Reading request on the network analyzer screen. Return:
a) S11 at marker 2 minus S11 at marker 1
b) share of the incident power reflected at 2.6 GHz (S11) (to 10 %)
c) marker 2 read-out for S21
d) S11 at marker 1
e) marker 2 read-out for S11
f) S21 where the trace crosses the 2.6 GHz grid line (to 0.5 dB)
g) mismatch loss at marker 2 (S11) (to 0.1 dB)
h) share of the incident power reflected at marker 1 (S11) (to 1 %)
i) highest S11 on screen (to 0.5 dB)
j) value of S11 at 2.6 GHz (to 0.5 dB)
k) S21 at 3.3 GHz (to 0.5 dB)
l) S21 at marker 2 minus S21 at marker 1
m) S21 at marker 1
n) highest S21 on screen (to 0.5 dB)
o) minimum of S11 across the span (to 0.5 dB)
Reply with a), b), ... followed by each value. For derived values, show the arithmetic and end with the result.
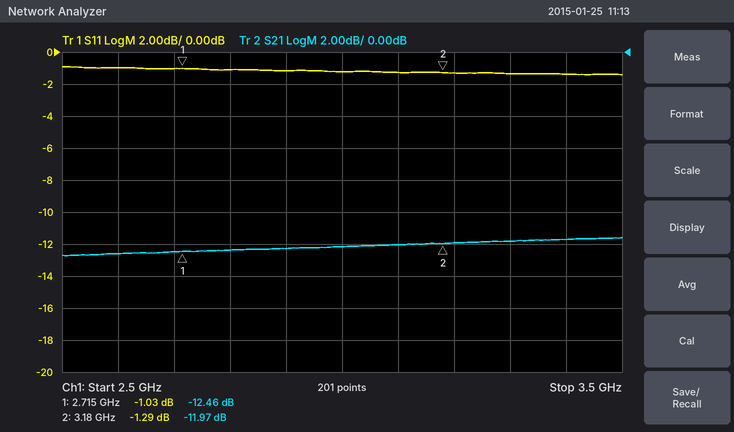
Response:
a) -1.29 − (-1.03) = -0.26 dB
b) 10^(-1/10) ≈ 79.4 %, so 80 % to the nearest 10 %
c) -11.97 dB
d) -1.03 dB
e) -1.29 dB
f) -12.5 dB
g) −10 log10(1 − 10^(-1.29/10)) ≈ 5.9 dB
h) 10^(-1.03/10) ≈ 79 %
i) -1.0 dB
j) -1.0 dB
k) -12.0 dB
l) -11.97 − (-12.46) = 0.49 dB
m) -12.46 dB
n) -11.5 dB
o) -1.5 dB
